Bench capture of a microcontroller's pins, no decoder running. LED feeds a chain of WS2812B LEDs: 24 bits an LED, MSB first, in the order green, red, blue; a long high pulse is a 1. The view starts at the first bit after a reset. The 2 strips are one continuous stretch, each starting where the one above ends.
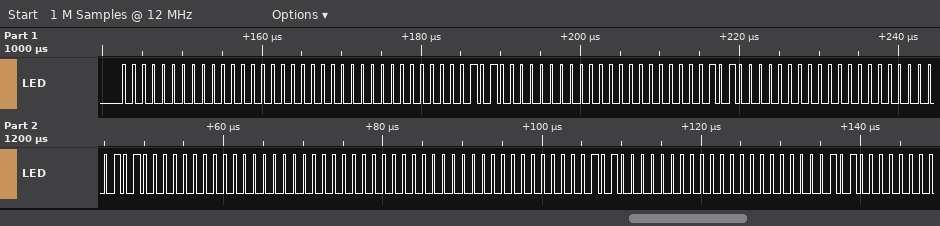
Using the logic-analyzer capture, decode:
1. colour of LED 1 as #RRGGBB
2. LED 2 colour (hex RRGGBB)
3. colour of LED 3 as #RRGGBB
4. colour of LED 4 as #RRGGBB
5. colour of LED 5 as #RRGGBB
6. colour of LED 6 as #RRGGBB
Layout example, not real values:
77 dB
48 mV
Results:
#000000
#140000
#140000
#140000
#000000
#140000
